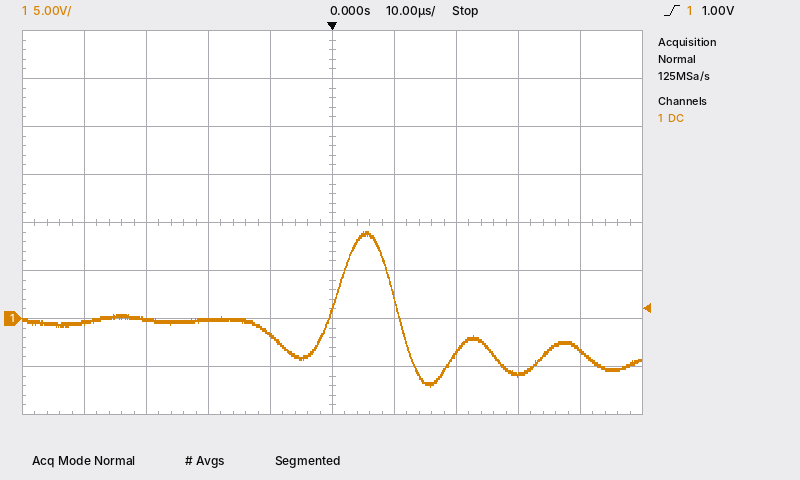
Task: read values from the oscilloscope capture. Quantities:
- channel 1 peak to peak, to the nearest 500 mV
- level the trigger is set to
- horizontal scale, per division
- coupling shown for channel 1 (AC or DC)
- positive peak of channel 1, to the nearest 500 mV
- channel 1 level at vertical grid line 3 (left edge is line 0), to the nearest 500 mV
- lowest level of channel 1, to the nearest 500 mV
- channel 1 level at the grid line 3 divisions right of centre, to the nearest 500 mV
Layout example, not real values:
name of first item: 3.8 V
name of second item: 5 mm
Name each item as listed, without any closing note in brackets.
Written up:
channel 1 peak to peak, to the nearest 500 mV: 16.0 V
level the trigger is set to: 1.00 V
horizontal scale, per division: 10 µs
coupling shown for channel 1: DC
positive peak of channel 1, to the nearest 500 mV: 9.0 V
channel 1 level at vertical grid line 3 (left edge is line 0), to the nearest 500 mV: 0.0 V
lowest level of channel 1, to the nearest 500 mV: -7.0 V
channel 1 level at the grid line 3 divisions right of centre, to the nearest 500 mV: -6.0 V
